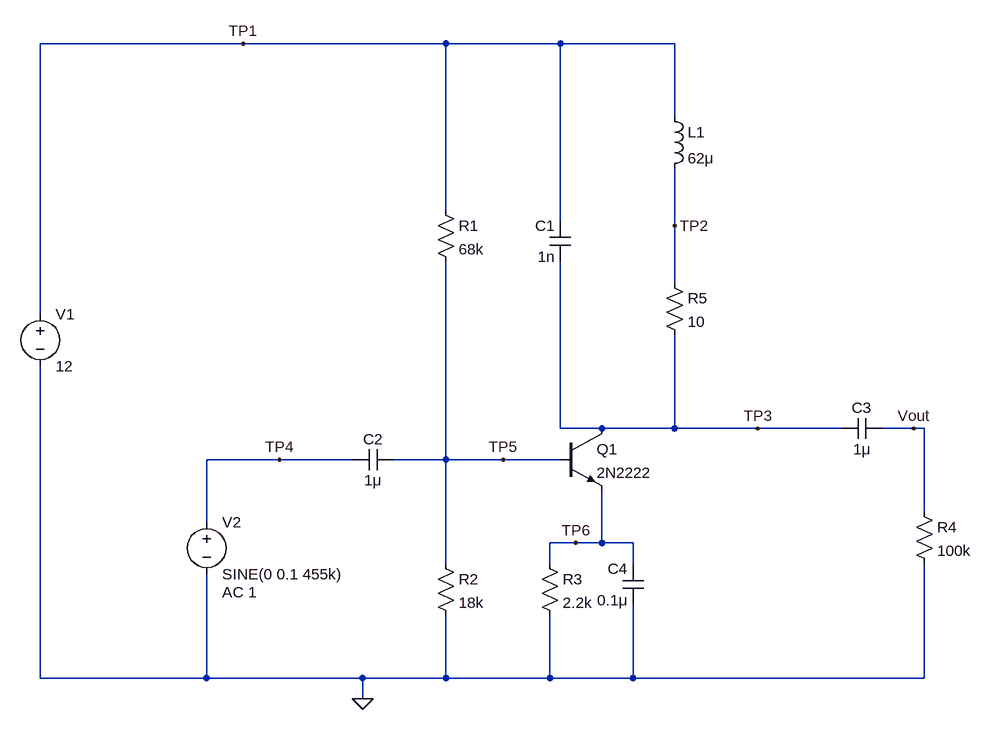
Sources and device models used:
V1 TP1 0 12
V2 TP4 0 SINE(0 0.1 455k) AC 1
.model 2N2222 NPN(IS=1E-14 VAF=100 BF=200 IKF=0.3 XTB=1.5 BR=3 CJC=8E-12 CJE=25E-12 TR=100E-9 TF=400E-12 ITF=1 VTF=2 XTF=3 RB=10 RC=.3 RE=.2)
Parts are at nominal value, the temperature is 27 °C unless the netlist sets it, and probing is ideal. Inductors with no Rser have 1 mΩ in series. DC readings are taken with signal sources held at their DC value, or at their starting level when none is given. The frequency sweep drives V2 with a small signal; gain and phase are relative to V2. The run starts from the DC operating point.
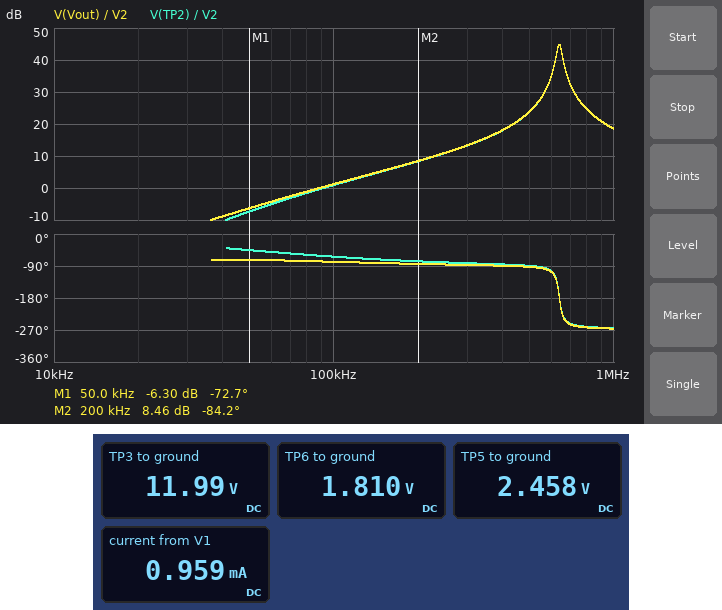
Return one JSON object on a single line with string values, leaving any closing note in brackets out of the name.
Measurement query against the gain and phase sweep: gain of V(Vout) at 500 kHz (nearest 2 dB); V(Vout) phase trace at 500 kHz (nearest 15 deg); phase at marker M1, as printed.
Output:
{"gain of V(Vout) at 500 kHz": "24 dB", "V(Vout) phase trace at 500 kHz": "-90 deg", "phase at marker M1, as printed": "-72.7 deg"}
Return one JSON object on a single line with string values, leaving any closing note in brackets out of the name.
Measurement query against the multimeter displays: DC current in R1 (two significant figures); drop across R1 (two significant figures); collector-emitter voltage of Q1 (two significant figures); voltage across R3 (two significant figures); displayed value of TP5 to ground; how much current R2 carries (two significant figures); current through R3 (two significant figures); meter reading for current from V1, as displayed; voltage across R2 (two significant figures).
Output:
{"DC current in R1": "140 µA", "drop across R1": "9.5 V", "collector-emitter voltage of Q1": "10 V", "voltage across R3": "1.8 V", "displayed value of TP5 to ground": "2.458 V", "how much current R2 carries": "140 µA", "current through R3": "820 µA", "meter reading for current from V1, as displayed": "0.959 mA", "voltage across R2": "2.5 V"}
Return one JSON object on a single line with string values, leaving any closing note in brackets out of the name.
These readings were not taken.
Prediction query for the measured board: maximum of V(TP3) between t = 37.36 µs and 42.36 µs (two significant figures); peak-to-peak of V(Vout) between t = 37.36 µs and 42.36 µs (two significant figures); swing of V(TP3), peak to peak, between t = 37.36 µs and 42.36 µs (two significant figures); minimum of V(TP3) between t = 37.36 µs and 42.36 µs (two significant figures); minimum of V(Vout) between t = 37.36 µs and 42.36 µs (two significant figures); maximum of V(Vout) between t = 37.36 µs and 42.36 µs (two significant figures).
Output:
{"maximum of V(TP3) between t = 37.36 µs and 42.36 µs": "13 V", "peak-to-peak of V(Vout) between t = 37.36 µs and 42.36 µs": "1.5 V", "swing of V(TP3), peak to peak, between t = 37.36 µs and 42.36 µs": "1.5 V", "minimum of V(TP3) between t = 37.36 µs and 42.36 µs": "11 V", "minimum of V(Vout) between t = 37.36 µs and 42.36 µs": "-710 mV", "maximum of V(Vout) between t = 37.36 µs and 42.36 µs": "780 mV"}
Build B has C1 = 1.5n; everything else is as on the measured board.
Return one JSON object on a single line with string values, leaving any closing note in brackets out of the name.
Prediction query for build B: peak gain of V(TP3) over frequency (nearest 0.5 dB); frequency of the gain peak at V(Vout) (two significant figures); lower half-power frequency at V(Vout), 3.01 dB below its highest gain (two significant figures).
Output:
{"peak gain of V(TP3) over frequency": "41.5 dB", "frequency of the gain peak at V(Vout)": "520 kHz", "lower half-power frequency at V(Vout), 3.01 dB below its highest gain": "510 kHz"}
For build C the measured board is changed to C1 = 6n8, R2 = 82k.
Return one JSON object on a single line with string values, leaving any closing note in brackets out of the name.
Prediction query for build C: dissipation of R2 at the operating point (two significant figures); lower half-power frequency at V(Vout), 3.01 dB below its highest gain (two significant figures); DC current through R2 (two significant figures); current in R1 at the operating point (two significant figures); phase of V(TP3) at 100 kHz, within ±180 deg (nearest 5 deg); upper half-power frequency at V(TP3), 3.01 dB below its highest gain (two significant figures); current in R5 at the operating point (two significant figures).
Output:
{"dissipation of R2 at the operating point": "460 µW", "lower half-power frequency at V(Vout), 3.01 dB below its highest gain": "230 kHz", "DC current through R2": "75 µA", "current in R1 at the operating point": "86 µA", "phase of V(TP3) at 100 kHz, within ±180 deg": "-50 deg", "upper half-power frequency at V(TP3), 3.01 dB below its highest gain": "260 kHz", "current in R5 at the operating point": "2.5 mA"}
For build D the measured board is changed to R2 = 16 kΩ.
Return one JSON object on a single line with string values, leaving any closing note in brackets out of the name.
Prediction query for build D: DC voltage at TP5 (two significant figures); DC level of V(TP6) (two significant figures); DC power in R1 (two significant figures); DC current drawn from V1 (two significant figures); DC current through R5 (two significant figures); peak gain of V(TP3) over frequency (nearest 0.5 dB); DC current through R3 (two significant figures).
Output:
{"DC voltage at TP5": "2.2 V", "DC level of V(TP6)": "1.6 V", "DC power in R1": "1.4 mW", "DC current drawn from V1": "870 µA", "DC current through R5": "720 µA", "peak gain of V(TP3) over frequency": "44.0 dB", "DC current through R3": "730 µA"}
